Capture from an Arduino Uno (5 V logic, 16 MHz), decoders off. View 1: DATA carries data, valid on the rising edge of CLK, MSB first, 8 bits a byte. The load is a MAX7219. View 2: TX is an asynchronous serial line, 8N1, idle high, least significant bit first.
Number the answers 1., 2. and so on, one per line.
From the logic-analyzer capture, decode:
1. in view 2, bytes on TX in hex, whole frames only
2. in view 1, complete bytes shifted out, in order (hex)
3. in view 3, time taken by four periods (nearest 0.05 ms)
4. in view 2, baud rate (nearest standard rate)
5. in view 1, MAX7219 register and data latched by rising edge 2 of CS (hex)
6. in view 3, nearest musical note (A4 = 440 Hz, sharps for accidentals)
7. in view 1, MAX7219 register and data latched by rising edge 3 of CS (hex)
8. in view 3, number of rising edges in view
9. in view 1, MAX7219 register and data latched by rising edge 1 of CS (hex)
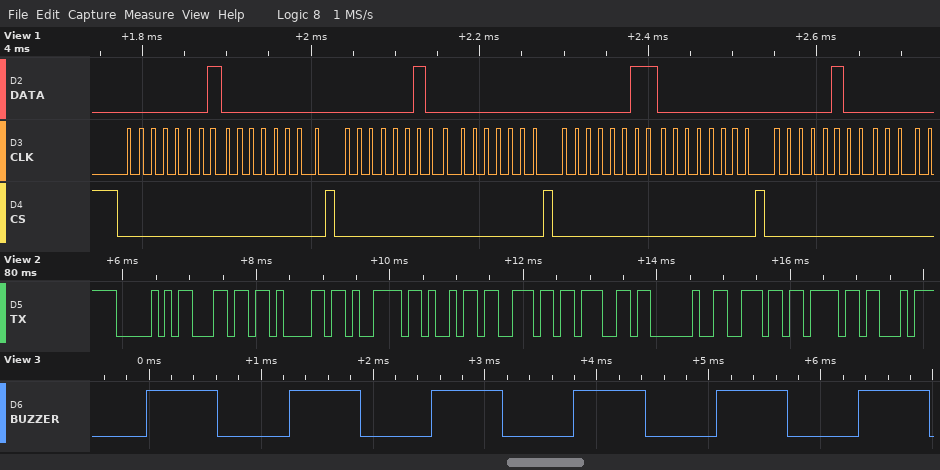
1. 50 6C 61 79 69 6E 67 20 6E 6F
2. 0x01 0x00 0x02 0x00 0x03 0x00 0x04
3. 5.10 ms
4. 9600 baud
5. register 0x2, data 0x00
6. G5
7. register 0x3, data 0x00
8. 6
9. register 0x1, data 0x00
